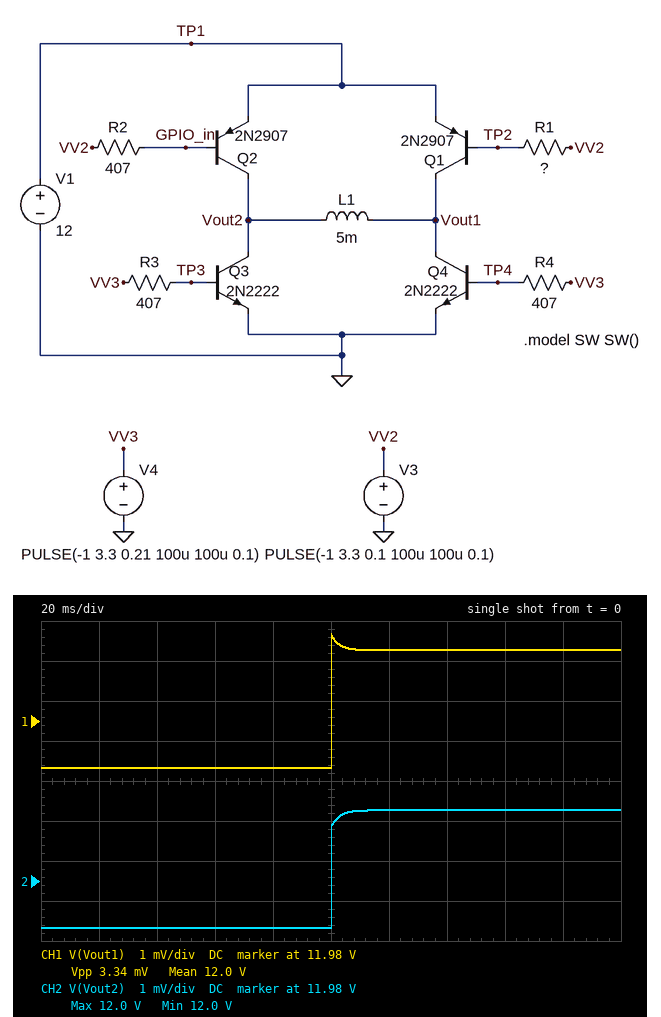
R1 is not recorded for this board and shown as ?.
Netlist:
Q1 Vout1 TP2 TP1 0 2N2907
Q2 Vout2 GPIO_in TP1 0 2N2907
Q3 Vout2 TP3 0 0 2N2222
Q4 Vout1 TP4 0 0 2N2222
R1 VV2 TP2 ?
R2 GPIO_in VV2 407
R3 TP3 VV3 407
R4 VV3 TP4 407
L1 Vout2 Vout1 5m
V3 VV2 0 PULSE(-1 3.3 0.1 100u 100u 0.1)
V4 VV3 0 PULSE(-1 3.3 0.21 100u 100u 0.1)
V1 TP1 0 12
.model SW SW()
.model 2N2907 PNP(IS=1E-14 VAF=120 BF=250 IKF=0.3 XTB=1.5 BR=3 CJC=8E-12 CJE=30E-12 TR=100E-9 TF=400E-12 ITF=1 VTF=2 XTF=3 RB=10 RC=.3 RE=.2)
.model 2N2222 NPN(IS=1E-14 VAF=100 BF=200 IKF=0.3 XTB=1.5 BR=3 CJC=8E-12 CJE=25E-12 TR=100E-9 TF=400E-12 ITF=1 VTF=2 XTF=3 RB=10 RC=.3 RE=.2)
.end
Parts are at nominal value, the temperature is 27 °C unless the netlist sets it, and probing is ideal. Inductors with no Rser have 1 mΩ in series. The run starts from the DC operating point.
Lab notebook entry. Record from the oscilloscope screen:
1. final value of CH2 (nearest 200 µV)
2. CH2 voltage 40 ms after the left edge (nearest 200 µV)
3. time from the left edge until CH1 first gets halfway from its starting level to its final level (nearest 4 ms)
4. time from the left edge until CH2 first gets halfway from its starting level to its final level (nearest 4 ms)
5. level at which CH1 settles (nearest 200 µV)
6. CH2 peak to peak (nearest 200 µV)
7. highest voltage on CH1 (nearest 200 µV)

11.9868 V
11.9838 V
100 ms
100 ms
11.9868 V
3.0 mV
11.9872 V
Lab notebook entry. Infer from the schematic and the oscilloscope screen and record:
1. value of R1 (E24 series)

330 Ω
